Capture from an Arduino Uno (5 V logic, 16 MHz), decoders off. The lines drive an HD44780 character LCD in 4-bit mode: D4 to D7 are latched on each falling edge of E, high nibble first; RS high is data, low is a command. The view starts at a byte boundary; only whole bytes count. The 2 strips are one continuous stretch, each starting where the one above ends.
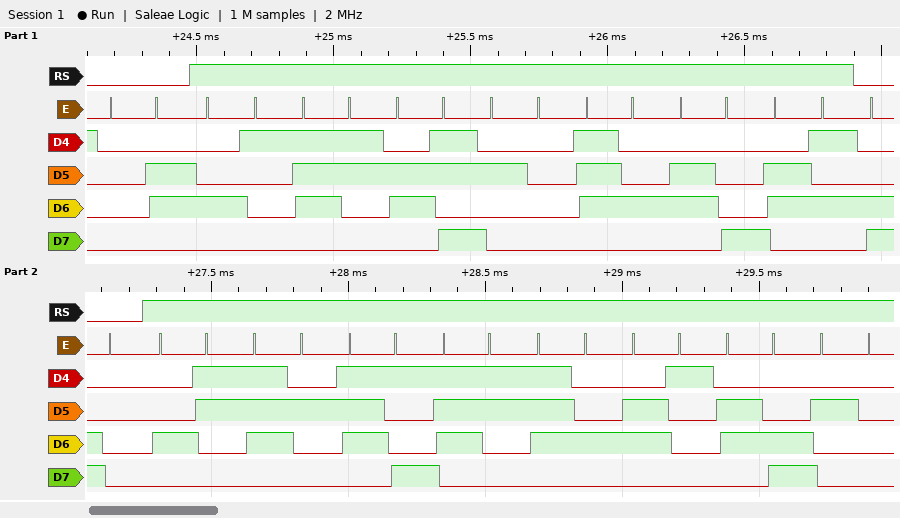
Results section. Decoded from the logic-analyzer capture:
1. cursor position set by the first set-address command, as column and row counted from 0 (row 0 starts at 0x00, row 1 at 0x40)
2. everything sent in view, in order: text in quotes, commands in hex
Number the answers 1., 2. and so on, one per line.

1. column 0, row 1
2. 0x06 "Ask the" 0xC0 "Crystal "
